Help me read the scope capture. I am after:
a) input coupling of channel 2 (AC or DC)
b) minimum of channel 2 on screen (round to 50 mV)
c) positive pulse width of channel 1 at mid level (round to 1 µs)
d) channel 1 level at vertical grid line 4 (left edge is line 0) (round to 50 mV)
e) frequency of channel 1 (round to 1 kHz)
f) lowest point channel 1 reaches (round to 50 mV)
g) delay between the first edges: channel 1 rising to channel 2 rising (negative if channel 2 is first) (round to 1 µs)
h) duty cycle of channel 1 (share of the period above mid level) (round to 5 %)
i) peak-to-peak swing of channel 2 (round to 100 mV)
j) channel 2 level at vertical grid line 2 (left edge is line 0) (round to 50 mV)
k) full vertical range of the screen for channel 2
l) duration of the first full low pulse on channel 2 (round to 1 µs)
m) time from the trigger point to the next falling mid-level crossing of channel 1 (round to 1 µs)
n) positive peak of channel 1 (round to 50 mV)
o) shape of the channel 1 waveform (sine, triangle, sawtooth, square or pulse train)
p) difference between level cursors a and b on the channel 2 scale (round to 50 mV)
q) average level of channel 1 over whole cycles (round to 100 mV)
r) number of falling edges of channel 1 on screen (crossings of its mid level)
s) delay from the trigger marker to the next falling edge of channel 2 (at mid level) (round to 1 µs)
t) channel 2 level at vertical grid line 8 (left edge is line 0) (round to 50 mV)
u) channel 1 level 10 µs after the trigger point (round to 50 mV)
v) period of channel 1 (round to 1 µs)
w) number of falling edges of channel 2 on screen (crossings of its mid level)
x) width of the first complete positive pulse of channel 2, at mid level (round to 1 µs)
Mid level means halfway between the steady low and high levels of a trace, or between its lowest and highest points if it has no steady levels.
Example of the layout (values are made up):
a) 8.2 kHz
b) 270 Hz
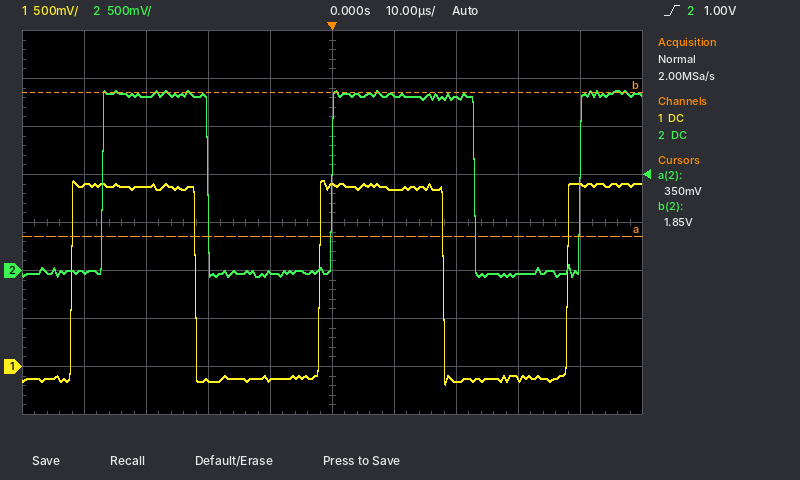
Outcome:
a) DC
b) -50 mV
c) 20 µs
d) -150 mV
e) 25 kHz
f) -200 mV
g) +5 µs
h) 50 %
i) 1.90 V
j) 1.80 V
k) 4 V
l) 20 µs
m) 18 µs
n) 1.95 V
o) square
p) 1.50 V
q) 900 mV
r) 2
s) 23 µs
t) -50 mV
u) 1.85 V
v) 40 µs
w) 2
x) 17 µs
